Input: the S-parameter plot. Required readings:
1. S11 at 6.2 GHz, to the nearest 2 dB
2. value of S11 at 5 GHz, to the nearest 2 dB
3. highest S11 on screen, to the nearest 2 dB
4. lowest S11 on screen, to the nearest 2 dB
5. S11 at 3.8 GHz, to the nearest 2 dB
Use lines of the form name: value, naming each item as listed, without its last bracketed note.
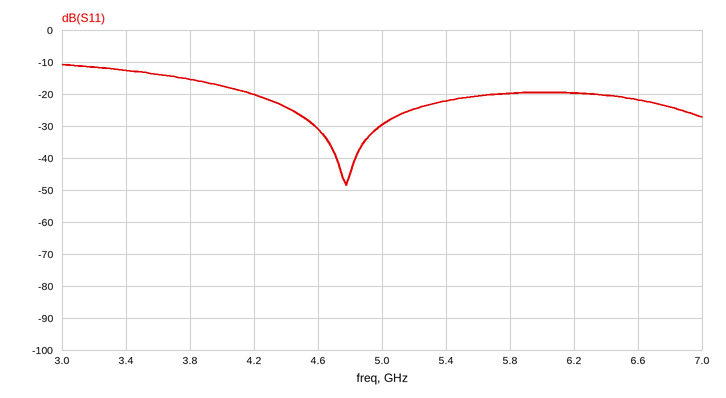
S11 at 6.2 GHz, to the nearest 2 dB: -20 dB
value of S11 at 5 GHz, to the nearest 2 dB: -30 dB
highest S11 on screen, to the nearest 2 dB: -10 dB
lowest S11 on screen, to the nearest 2 dB: -48 dB
S11 at 3.8 GHz, to the nearest 2 dB: -16 dB
